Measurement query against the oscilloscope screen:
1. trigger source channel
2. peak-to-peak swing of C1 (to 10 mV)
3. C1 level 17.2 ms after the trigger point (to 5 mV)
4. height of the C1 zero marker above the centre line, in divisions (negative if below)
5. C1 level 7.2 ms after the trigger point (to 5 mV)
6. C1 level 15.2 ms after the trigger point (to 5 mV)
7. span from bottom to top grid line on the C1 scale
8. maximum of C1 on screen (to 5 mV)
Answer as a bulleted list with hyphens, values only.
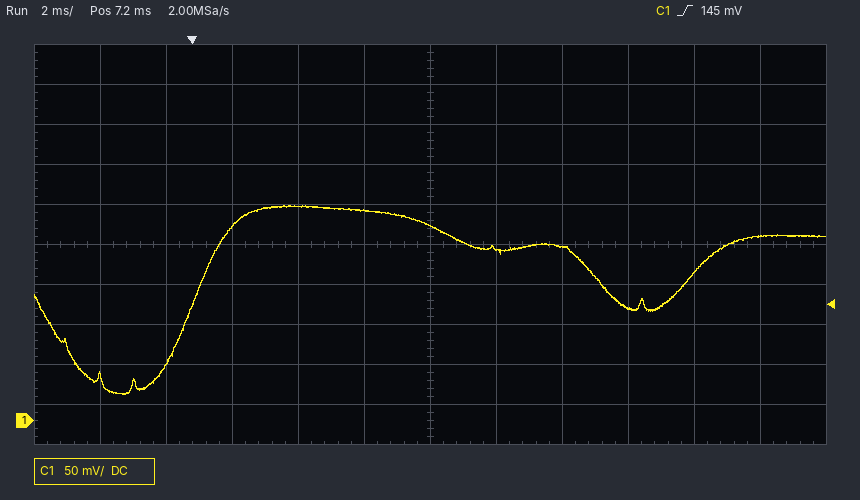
- C1
- 240 mV
- 230 mV
- -4.4 div
- 245 mV
- 185 mV
- 500 mV
- 270 mV
